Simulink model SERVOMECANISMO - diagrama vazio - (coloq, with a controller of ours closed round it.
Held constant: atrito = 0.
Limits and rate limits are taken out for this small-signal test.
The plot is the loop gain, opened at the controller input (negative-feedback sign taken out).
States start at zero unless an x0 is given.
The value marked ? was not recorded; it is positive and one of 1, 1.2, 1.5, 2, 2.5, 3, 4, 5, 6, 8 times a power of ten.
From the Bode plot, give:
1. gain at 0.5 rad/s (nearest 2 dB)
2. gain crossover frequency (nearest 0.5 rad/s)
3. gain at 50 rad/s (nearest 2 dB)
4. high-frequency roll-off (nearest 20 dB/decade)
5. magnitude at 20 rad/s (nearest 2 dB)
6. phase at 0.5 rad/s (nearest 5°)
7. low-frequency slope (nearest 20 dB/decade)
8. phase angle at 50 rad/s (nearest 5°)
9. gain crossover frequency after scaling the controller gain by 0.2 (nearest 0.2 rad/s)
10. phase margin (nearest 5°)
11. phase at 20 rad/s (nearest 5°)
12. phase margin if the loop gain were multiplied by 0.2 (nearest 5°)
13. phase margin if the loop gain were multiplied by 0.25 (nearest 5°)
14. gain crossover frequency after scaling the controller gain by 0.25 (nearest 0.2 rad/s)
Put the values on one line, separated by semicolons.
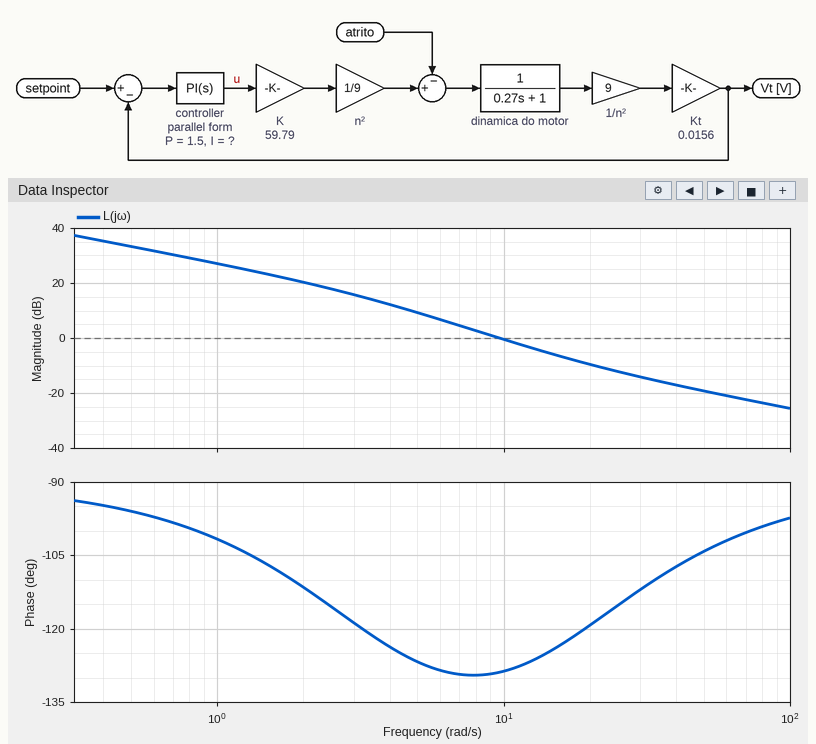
34 dB; 9.5 rad/s; -20 dB; -20 dB/decade; -10 dB; -95°; -20 dB/decade; -105°; 3.4 rad/s; 50°; -120°; 60°; 55°; 4.0 rad/s
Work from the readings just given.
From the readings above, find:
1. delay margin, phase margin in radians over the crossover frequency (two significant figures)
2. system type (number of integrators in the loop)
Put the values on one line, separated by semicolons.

0.092 s; 1
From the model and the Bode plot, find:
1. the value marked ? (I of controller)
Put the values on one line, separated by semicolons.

25
